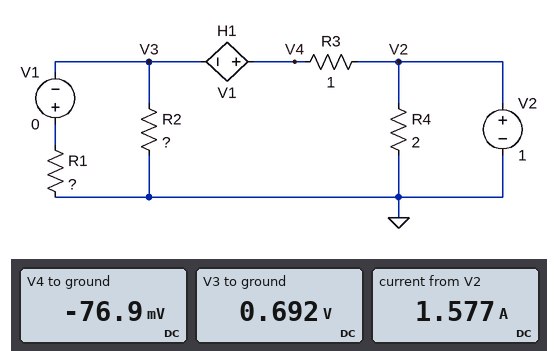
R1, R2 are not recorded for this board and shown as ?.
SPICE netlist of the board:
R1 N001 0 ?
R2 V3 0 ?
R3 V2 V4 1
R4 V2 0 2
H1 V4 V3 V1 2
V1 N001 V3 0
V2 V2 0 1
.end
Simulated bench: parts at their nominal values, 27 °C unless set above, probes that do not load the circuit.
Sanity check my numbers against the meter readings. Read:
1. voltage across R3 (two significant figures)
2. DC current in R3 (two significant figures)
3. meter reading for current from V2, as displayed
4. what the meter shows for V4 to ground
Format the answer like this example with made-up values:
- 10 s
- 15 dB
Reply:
- 1.1 V
- 1.1 A
- 1.577 A
- -76.9 mV
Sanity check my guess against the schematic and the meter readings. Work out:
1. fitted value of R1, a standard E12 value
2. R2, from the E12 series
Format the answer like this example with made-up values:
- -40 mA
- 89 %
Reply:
- 1.8 Ω
- 1 Ω
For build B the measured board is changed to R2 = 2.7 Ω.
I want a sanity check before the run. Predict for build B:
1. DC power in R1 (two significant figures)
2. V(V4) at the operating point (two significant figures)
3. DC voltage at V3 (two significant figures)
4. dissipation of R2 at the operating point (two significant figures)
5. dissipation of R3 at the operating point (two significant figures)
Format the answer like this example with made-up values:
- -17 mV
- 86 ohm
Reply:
- 840 mW
- -140 mV
- 1.2 V
- 560 mW
- 1.3 W
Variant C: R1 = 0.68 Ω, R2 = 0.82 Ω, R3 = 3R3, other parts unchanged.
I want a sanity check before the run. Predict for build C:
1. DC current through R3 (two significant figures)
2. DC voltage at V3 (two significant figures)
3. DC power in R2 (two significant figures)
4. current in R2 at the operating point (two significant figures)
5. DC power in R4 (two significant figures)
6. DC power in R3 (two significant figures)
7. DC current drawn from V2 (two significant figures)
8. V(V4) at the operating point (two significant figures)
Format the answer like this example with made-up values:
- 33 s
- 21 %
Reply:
- 390 mA
- 140 mV
- 25 mW
- 180 mA
- 500 mW
- 500 mW
- 890 mA
- -280 mV
